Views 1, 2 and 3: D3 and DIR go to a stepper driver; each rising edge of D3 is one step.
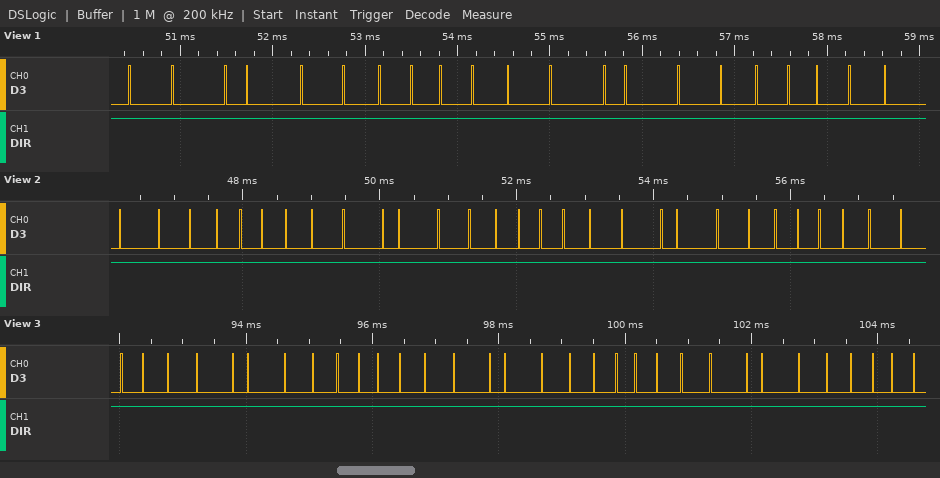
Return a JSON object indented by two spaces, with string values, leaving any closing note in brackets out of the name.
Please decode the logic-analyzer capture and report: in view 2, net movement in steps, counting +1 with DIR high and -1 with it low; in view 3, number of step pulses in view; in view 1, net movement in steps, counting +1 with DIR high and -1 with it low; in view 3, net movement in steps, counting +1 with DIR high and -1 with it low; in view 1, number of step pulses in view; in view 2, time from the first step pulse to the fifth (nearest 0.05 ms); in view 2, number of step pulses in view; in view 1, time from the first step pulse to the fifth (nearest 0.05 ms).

{
  "in view 2, net movement in steps, counting +1 with DIR high and -1 with it low": "+29",
  "in view 3, number of step pulses in view": "32",
  "in view 1, net movement in steps, counting +1 with DIR high and -1 with it low": "+21",
  "in view 3, net movement in steps, counting +1 with DIR high and -1 with it low": "+32",
  "in view 1, number of step pulses in view": "21",
  "in view 2, time from the first step pulse to the fifth": "1.75 ms",
  "in view 2, number of step pulses in view": "29",
  "in view 1, time from the first step pulse to the fifth": "1.85 ms"
}
